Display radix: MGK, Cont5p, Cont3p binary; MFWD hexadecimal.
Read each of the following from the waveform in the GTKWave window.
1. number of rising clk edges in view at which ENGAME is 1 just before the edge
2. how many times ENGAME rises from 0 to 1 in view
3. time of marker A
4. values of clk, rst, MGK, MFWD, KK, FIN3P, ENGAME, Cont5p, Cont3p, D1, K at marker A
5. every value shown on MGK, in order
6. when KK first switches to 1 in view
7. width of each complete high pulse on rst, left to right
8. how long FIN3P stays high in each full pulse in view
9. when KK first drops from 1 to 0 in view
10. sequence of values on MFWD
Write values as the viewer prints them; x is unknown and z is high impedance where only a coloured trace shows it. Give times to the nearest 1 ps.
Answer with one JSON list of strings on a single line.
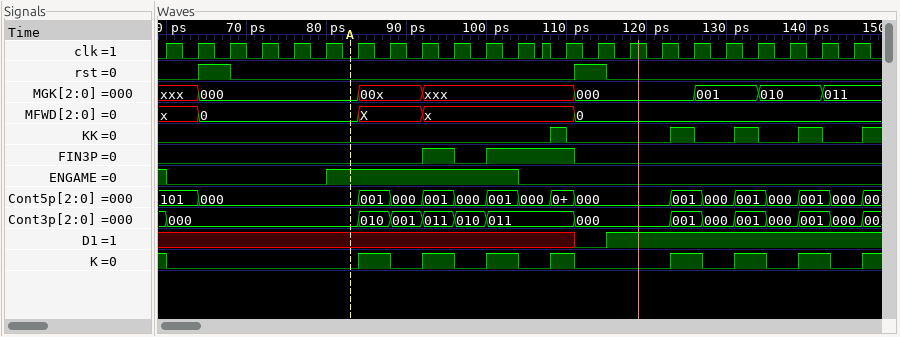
["7", "1", "83 ps", "clk=0, rst=0, MGK=000, MFWD=0, KK=0, FIN3P=0, ENGAME=1, Cont5p=000, Cont3p=000, D1=x, K=0", "xxx, 000, 00x, xxx, 000, 001, 010, 011", "108 ps", "4 ps, 4 ps", "4 ps, 11 ps", "110 ps", "x, 0, X, x, 0"]
